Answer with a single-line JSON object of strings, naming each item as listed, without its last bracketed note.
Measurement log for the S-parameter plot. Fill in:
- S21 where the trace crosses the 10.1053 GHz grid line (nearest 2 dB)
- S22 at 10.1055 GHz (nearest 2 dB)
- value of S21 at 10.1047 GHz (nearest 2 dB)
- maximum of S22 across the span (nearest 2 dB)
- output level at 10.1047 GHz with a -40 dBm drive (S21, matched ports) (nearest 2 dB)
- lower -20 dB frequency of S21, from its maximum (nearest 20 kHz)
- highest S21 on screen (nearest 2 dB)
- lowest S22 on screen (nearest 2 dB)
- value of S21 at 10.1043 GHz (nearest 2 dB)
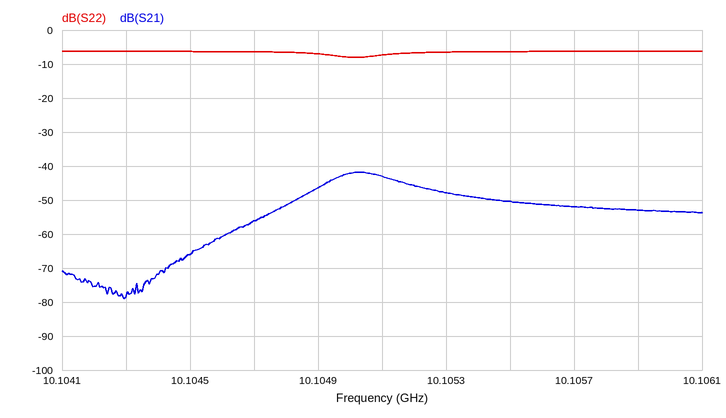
{"S21 where the trace crosses the 10.1053 GHz grid line": "-48 dB", "S22 at 10.1055 GHz": "-6 dB", "value of S21 at 10.1047 GHz": "-56 dB", "maximum of S22 across the span": "-6 dB", "output level at 10.1047 GHz with a -40 dBm drive (S21, matched ports)": "-96 dBm", "lower -20 dB frequency of S21, from its maximum": "10.10458 GHz", "highest S21 on screen": "-42 dB", "lowest S22 on screen": "-8 dB", "value of S21 at 10.1043 GHz": "-78 dB"}
